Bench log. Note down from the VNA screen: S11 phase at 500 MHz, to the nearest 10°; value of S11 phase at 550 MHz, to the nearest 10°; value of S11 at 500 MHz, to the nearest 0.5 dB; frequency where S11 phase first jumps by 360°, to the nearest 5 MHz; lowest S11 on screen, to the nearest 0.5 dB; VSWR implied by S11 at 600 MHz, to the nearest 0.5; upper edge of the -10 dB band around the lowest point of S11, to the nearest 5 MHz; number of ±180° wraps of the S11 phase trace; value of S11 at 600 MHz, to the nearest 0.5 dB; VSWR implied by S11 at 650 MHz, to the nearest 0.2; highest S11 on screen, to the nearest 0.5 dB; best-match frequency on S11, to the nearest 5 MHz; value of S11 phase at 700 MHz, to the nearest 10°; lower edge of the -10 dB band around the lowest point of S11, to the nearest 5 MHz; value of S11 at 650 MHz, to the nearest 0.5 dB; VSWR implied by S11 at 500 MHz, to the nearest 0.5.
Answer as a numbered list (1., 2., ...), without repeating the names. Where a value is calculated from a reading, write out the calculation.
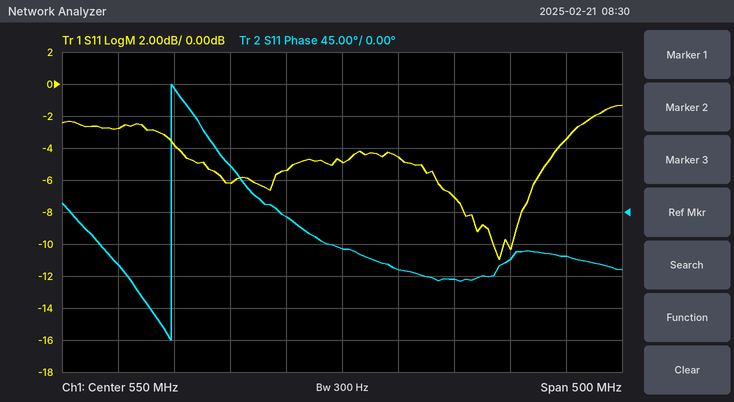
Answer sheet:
1. -10°
2. -50°
3. -5.5 dB
4. 400 MHz
5. -11.0 dB
6. |Γ| = 10^(-4.5/20) = 0.5957; VSWR = (1 + 0.5957)/(1 − 0.5957) ≈ 4.0
7. 695 MHz
8. 1
9. -4.5 dB
10. |Γ| = 10^(-7/20) = 0.4467; VSWR = (1 + 0.4467)/(1 − 0.4467) ≈ 2.6
11. -1.5 dB
12. 690 MHz
13. -70°
14. 685 MHz
15. -7.0 dB
16. |Γ| = 10^(-5.5/20) = 0.5309; VSWR = (1 + 0.5309)/(1 − 0.5309) ≈ 3.26, so 3.5 to the nearest 0.5
